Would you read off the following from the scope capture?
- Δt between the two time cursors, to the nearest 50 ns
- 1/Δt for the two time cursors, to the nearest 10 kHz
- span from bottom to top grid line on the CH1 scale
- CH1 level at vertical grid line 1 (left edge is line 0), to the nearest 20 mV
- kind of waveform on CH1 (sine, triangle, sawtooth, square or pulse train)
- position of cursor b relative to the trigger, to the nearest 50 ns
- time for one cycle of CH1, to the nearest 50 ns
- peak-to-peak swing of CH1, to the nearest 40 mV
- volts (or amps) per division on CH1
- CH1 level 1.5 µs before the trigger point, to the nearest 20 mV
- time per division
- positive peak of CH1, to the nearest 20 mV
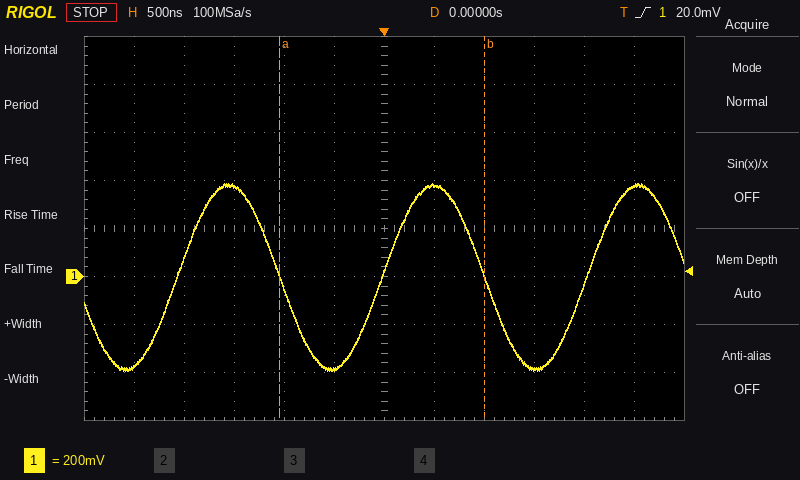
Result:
2.05 µs
490 kHz
1.6 V
-380 mV
sine
+1.00 µs
2.05 µs
760 mV
200 mV
380 mV
500 ns
380 mV
